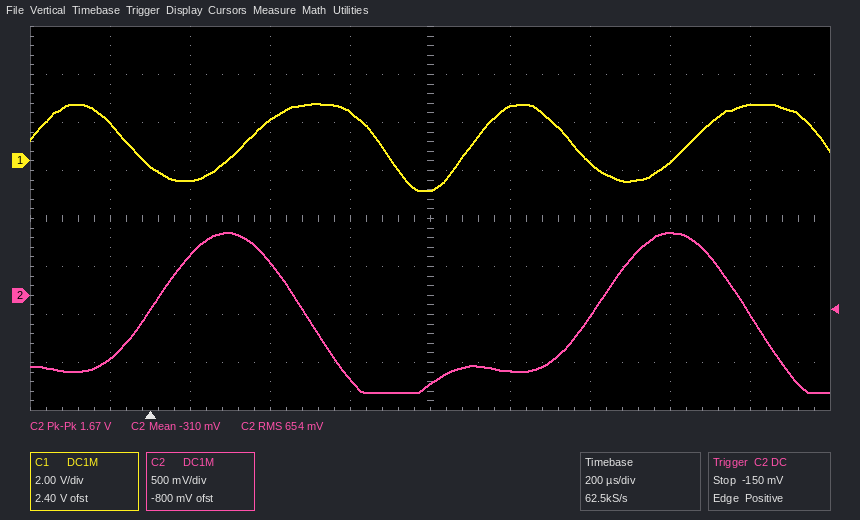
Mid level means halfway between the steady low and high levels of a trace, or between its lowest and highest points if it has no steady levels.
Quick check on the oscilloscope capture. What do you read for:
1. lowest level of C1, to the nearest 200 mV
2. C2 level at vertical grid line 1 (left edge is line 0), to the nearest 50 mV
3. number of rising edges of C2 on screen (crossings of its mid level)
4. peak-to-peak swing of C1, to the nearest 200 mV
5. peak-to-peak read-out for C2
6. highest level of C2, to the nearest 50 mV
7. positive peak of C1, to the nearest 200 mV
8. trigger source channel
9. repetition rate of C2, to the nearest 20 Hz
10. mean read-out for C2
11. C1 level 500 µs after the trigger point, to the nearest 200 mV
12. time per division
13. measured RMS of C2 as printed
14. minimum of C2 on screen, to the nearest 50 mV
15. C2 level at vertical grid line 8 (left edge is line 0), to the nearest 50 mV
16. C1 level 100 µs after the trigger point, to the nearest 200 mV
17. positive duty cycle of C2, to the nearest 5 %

-1.2 V
-650 mV
2
3.6 V
1.67 V
650 mV
2.4 V
C2
900 Hz
-310 mV
2.0 V
200 µs
654 mV
-1.00 V
650 mV
-800 mV
35 %
